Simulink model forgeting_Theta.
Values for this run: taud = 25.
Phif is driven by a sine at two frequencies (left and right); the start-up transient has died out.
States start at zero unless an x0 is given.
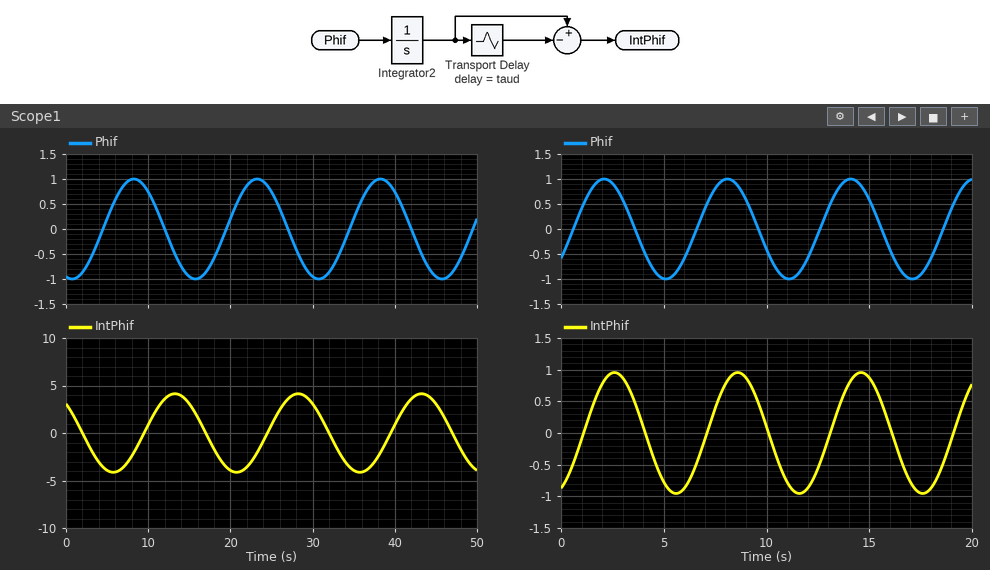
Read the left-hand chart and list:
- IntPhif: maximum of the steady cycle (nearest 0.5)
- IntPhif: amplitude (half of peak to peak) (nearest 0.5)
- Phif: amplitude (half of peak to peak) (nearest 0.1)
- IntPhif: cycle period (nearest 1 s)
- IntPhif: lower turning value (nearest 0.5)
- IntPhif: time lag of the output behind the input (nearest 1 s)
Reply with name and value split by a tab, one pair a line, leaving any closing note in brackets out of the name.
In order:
IntPhif: maximum of the steady cycle	4.0
IntPhif: amplitude (half of peak to peak)	4.0
Phif: amplitude (half of peak to peak)	1.0
IntPhif: cycle period	15 s
IntPhif: lower turning value	-4.0
IntPhif: time lag of the output behind the input	5 s
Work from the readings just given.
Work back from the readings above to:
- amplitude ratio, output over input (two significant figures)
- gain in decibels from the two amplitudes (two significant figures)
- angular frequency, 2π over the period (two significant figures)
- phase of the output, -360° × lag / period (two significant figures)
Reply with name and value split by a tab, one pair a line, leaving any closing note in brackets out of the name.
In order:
amplitude ratio, output over input	4.0
gain in decibels from the two amplitudes	12 dB
angular frequency, 2π over the period	0.42 rad/s
phase of the output, -360° × lag / period	-120°
